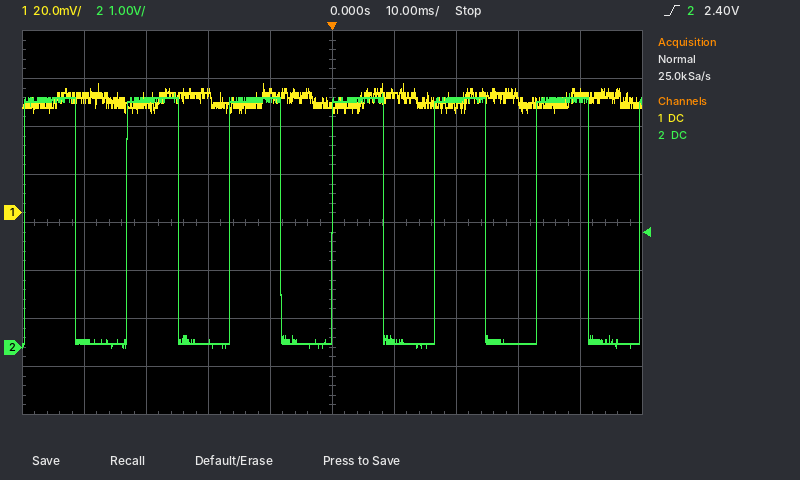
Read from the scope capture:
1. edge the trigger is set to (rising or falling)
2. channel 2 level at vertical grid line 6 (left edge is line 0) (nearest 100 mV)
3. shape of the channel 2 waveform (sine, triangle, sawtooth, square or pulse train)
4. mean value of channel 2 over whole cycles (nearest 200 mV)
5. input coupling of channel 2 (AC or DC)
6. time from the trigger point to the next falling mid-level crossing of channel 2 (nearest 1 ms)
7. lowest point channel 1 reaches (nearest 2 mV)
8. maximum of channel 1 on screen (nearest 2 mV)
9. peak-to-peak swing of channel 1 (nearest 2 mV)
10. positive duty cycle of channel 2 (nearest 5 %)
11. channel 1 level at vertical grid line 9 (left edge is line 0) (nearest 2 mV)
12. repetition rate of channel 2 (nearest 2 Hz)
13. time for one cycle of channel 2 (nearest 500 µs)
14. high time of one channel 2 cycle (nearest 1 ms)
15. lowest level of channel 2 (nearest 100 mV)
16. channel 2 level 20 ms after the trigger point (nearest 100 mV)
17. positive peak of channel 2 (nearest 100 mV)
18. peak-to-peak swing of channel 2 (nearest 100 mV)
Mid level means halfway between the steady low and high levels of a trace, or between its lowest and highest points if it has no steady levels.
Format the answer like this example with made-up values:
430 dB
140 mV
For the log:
rising
100 mV
square
2.6 V
DC
8 ms
42 mV
54 mV
12 mV
50 %
50 mV
60 Hz
16.5 ms
8 ms
0.0 V
5.2 V
5.3 V
5.3 V
